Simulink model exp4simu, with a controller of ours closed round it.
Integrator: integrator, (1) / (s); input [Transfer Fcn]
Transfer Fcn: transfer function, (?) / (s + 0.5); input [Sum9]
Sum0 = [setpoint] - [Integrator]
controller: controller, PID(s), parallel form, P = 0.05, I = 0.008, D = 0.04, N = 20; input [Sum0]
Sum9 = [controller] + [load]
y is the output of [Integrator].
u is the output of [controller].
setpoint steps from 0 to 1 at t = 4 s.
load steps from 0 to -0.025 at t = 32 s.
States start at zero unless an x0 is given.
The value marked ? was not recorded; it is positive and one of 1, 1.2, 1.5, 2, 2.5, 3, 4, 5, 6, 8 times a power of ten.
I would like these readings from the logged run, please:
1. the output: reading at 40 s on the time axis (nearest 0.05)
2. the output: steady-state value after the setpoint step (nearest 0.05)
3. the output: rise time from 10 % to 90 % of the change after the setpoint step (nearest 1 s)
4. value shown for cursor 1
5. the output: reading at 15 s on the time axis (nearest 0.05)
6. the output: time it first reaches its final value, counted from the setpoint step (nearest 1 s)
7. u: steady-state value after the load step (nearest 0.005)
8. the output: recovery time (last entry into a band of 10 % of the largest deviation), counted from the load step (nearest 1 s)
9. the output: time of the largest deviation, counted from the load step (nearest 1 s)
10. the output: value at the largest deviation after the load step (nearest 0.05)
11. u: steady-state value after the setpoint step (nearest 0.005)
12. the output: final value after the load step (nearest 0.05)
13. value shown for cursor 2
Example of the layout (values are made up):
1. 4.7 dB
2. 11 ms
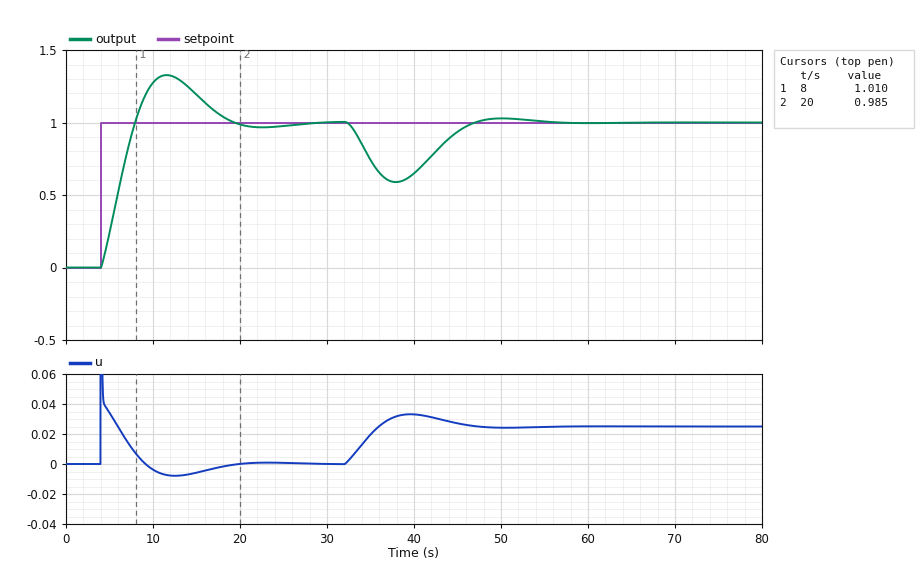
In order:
1. 0.65
2. 1.00
3. 3 s
4. 1.010
5. 1.20
6. 4 s
7. 0.025
8. 14 s
9. 6 s
10. 0.60
11. 0.000
12. 1.00
13. 0.985
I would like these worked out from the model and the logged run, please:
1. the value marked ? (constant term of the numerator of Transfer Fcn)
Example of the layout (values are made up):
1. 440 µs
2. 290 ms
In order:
1. 5
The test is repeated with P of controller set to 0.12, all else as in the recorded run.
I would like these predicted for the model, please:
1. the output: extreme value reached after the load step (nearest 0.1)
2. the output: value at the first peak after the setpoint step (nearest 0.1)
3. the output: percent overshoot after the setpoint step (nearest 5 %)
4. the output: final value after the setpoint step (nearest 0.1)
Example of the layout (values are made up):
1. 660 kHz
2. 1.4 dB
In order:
1. 0.8
2. 1.3
3. 30 %
4. 1.0
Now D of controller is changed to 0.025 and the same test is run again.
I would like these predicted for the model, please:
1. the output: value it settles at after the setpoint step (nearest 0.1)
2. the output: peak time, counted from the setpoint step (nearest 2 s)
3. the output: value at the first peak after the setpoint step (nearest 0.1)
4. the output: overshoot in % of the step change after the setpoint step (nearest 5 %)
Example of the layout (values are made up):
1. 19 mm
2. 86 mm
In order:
1. 1.0
2. 8 s
3. 1.4
4. 40 %
